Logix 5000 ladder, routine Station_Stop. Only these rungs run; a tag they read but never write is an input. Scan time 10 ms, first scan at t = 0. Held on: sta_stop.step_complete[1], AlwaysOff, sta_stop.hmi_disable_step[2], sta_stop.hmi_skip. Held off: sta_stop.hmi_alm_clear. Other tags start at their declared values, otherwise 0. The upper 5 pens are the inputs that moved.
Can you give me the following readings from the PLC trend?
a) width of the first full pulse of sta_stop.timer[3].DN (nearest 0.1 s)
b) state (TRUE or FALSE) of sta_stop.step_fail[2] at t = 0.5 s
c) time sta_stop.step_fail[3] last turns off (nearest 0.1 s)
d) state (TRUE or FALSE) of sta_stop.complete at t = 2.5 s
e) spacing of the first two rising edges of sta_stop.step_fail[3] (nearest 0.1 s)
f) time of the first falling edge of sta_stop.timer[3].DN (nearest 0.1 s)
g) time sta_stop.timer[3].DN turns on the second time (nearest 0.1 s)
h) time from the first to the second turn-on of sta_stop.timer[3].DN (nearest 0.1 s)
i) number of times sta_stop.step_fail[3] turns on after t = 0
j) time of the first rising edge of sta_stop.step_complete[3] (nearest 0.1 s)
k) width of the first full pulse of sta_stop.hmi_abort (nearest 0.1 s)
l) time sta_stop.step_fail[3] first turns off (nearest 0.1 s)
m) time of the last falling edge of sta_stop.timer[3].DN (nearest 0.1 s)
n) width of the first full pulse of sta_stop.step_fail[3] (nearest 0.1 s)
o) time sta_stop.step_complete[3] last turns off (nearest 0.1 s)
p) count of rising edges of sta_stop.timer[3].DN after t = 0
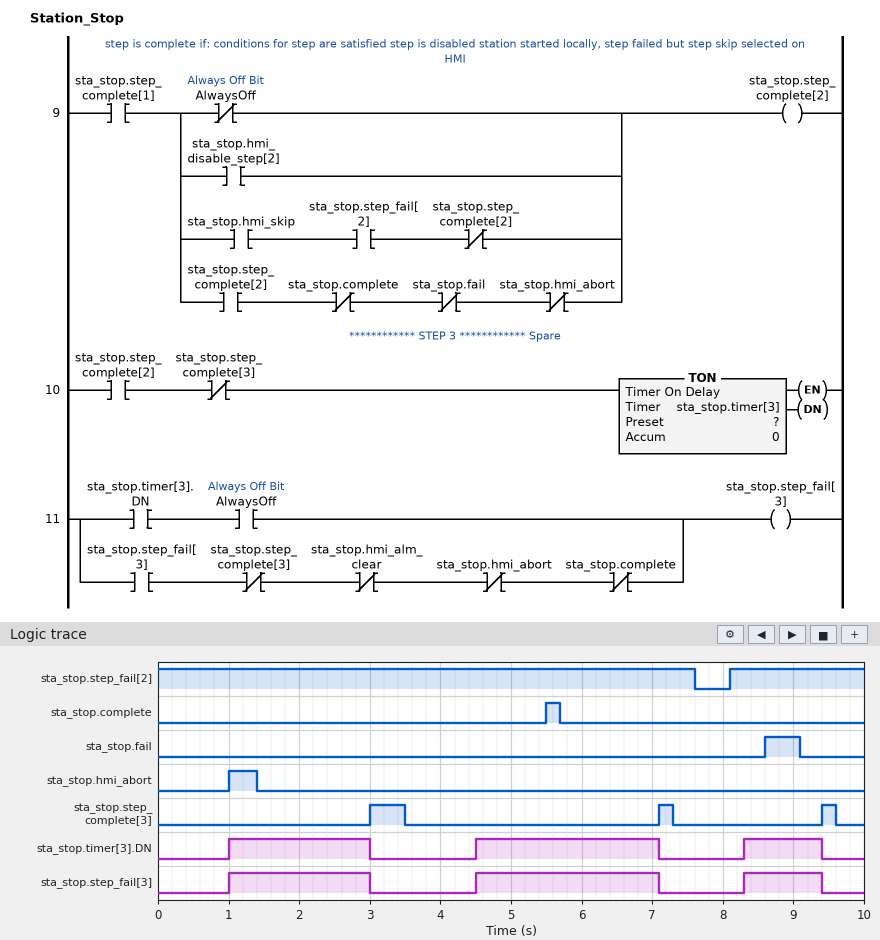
2.0 s
TRUE
9.4 s
FALSE
3.5 s
3.0 s
4.5 s
3.5 s
3
3.0 s
0.4 s
3.0 s
9.4 s
2.0 s
9.6 s
3
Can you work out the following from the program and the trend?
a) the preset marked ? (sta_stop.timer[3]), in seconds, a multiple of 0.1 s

1.0 s
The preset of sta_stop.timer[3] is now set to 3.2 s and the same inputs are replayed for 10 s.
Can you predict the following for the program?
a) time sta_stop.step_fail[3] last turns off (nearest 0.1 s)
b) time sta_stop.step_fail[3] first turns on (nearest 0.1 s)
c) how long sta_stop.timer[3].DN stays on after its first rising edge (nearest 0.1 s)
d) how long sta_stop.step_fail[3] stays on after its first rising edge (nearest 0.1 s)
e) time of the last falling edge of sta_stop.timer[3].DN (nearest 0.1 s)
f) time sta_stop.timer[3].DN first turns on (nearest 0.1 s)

7.1 s
6.7 s
0.4 s
0.4 s
7.1 s
6.7 s
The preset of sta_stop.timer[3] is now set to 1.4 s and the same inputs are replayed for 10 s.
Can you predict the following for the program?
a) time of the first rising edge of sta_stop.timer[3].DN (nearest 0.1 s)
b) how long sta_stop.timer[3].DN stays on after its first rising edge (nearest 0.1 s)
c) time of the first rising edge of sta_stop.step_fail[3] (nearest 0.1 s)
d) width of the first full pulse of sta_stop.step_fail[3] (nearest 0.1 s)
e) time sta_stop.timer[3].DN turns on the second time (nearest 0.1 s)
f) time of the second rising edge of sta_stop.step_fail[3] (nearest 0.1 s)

1.4 s
1.6 s
1.4 s
1.6 s
4.9 s
4.9 s
